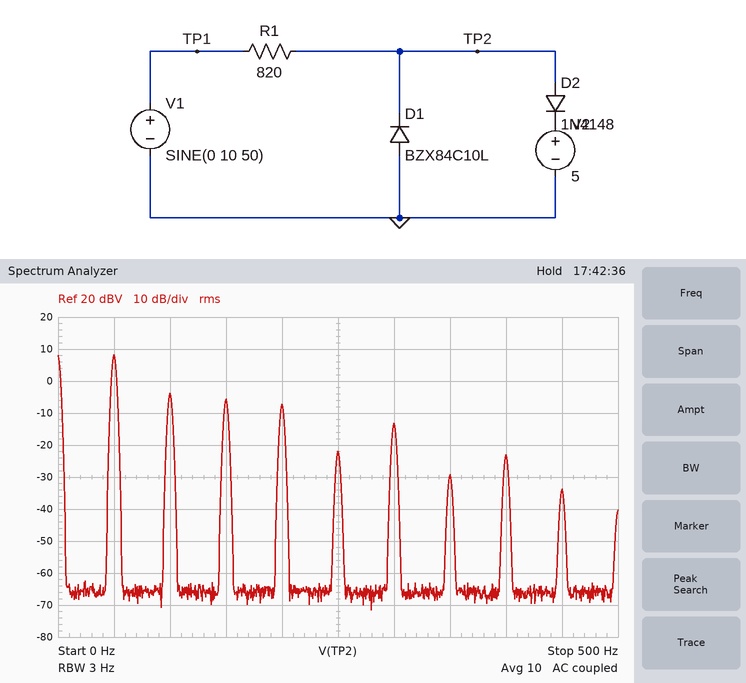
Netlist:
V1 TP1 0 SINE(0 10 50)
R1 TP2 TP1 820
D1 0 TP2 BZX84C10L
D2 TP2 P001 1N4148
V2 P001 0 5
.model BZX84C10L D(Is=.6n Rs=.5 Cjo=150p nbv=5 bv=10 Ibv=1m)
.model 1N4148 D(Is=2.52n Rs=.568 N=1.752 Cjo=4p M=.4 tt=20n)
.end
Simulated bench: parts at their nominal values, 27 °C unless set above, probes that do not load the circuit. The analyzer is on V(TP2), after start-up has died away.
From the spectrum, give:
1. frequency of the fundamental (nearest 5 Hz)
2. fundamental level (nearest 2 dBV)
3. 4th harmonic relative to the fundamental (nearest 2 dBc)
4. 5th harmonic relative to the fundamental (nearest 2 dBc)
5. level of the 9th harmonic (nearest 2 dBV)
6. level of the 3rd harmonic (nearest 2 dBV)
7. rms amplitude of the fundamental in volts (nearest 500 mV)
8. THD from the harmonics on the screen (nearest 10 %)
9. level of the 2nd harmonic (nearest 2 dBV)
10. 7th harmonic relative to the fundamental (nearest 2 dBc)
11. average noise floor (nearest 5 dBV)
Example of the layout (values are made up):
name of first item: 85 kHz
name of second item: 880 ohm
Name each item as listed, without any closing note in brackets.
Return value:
frequency of the fundamental: 50 Hz
fundamental level: 8 dBV
4th harmonic relative to the fundamental: -16 dBc
5th harmonic relative to the fundamental: -30 dBc
level of the 9th harmonic: -34 dBV
level of the 3rd harmonic: -6 dBV
rms amplitude of the fundamental in volts: 2.5 V
THD from the harmonics on the screen: 40 %
level of the 2nd harmonic: -4 dBV
7th harmonic relative to the fundamental: -38 dBc
average noise floor: -65 dBV
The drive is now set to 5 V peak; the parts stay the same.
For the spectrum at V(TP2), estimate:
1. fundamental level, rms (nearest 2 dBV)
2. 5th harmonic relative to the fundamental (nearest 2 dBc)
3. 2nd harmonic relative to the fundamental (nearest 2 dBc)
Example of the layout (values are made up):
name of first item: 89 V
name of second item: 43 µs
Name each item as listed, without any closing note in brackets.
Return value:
fundamental level, rms: 6 dBV
5th harmonic relative to the fundamental: -36 dBc
2nd harmonic relative to the fundamental: -8 dBc
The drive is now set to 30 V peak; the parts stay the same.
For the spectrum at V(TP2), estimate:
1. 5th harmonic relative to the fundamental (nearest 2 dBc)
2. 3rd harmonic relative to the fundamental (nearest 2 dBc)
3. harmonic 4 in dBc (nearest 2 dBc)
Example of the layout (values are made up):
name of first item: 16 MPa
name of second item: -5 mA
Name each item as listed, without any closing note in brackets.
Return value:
5th harmonic relative to the fundamental: -16 dBc
3rd harmonic relative to the fundamental: -10 dBc
harmonic 4 in dBc: -22 dBc
